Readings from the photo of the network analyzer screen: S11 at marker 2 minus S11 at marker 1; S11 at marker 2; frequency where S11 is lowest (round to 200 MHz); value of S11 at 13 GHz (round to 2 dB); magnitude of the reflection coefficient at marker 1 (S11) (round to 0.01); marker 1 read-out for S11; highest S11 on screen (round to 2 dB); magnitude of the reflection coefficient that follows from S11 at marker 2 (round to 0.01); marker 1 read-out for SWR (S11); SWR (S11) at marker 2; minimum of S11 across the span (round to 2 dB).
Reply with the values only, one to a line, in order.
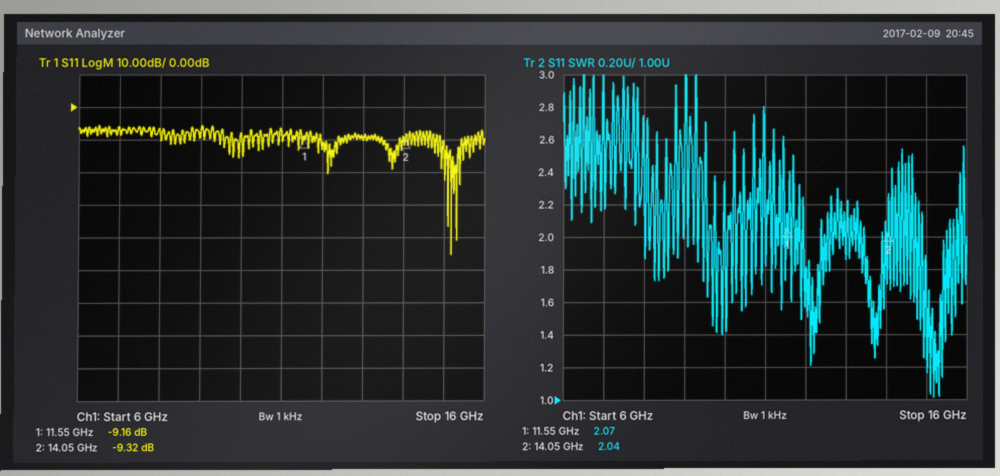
-0.16 dB
-9.32 dB
15.2 GHz
-10 dB
0.35
-9.16 dB
-6 dB
0.34
2.07
2.04
-46 dB
